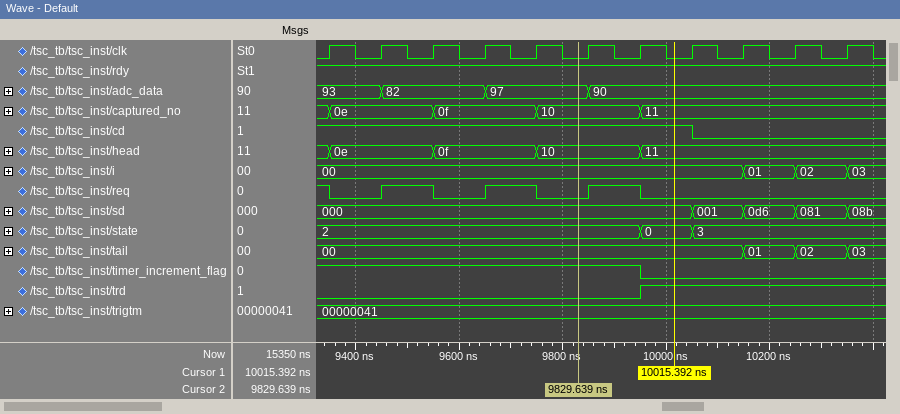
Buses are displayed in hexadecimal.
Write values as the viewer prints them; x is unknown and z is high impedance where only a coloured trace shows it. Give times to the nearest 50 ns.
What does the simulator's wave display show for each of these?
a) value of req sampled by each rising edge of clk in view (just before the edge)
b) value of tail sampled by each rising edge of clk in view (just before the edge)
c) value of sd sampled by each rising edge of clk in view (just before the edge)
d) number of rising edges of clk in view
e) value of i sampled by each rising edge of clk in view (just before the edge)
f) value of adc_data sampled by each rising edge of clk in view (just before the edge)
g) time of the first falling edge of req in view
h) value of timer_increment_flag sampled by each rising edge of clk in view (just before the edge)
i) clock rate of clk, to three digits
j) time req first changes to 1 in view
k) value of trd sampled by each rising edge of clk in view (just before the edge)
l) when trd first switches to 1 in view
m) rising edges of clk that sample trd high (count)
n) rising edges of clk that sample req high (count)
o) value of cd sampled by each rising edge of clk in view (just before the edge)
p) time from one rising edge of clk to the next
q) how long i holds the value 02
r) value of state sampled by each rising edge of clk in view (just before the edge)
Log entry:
1 0 1 0 1 0 1 0 0 0 0
00, 00, 00, 00, 00, 00, 00, 00, 00, 01, 02
000, 000, 000, 000, 000, 000, 000, 000, 001, 0d6, 081
11
00, 00, 00, 00, 00, 00, 00, 00, 00, 01, 02
93, 93, 82, 82, 97, 97, 90, 90, 90, 90, 90
9350 ns
1 1 1 1 1 1 1 0 0 0 0
10.0 MHz
9450 ns
0 0 0 0 0 0 0 1 1 1 1
9950 ns
4
4
1 1 1 1 1 1 1 1 0 0 0
100 ns
100 ns
2, 2, 2, 2, 2, 2, 2, 0, 3, 3, 3
